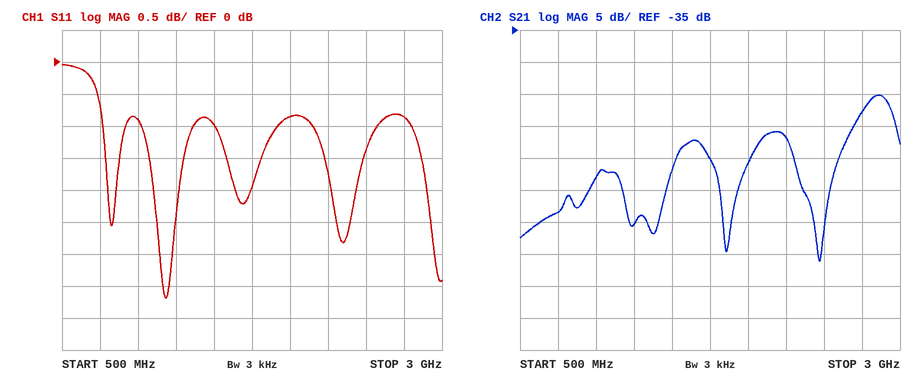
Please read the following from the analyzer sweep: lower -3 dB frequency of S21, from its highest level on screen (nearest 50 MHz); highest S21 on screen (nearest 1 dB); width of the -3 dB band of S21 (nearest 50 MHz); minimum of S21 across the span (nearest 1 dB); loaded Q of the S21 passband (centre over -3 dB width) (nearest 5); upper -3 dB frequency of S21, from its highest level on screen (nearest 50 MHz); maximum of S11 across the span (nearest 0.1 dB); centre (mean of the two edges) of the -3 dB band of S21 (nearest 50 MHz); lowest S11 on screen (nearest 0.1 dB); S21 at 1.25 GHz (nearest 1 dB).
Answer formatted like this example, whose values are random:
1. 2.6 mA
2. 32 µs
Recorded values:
1. 2.75 GHz
2. -45 dB
3. 200 MHz
4. -71 dB
5. 15
6. 2.95 GHz
7. 0.0 dB
8. 2.85 GHz
9. -3.7 dB
10. -65 dB
